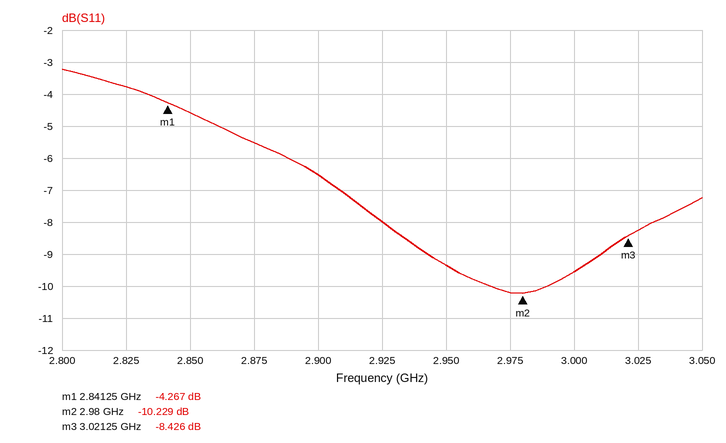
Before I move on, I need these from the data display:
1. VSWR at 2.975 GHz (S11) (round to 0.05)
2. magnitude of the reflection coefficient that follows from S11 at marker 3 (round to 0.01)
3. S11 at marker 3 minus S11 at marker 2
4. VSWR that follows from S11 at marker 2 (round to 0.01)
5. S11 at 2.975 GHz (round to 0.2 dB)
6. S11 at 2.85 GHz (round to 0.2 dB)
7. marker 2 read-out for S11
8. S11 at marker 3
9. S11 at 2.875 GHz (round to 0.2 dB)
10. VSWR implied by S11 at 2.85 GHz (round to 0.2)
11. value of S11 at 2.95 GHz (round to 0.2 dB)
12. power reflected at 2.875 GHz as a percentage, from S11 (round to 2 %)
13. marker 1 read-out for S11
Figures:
1.90
0.38
1.803 dB
1.89
-10.2 dB
-4.6 dB
-10.229 dB
-8.426 dB
-5.6 dB
3.8
-9.4 dB
28 %
-4.267 dB
